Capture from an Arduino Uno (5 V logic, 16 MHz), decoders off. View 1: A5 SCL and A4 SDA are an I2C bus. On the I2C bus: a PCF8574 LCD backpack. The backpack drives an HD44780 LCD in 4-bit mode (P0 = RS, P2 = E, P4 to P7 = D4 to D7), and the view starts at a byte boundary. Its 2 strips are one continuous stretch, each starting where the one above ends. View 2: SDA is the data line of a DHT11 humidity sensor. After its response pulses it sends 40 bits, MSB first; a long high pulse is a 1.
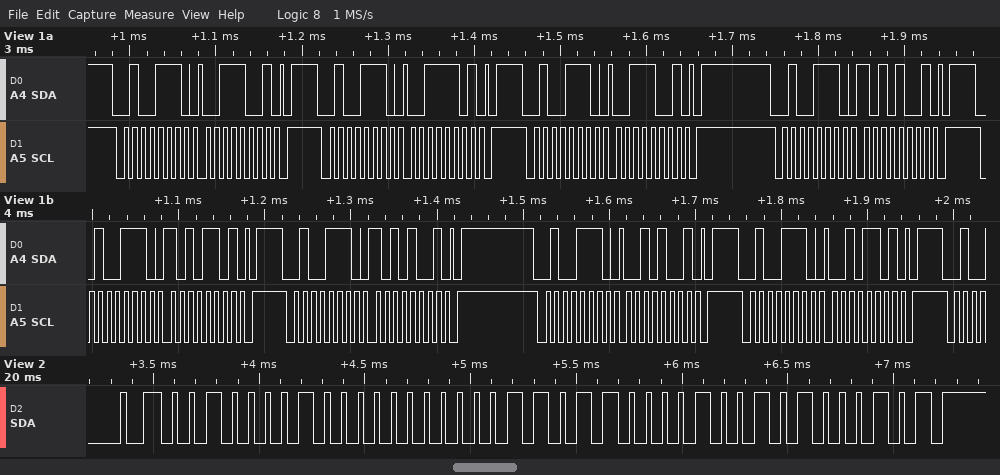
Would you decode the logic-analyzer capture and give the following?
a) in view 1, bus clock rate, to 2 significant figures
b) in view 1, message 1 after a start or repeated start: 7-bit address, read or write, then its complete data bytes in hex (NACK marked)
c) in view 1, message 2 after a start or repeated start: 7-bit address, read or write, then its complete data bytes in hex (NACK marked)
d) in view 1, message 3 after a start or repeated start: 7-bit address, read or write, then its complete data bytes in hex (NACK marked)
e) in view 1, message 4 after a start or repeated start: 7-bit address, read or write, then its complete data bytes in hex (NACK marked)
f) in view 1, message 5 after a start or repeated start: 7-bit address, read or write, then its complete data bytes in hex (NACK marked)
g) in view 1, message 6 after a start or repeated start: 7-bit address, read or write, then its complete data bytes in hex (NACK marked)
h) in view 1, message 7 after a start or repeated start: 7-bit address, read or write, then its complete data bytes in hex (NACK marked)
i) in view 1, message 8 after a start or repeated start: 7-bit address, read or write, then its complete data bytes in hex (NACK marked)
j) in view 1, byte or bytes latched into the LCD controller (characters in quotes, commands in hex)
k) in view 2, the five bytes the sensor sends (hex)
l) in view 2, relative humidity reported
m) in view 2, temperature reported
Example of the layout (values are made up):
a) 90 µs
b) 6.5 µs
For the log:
a) 100 kHz
b) 0x27 write: 39
c) 0x27 write: 3D
d) 0x27 write: 39
e) 0x27 write: A9
f) 0x27 write: AD
g) 0x27 write: A9
h) 0x27 write: 29
i) 0x27 write: 2D
j) ':'
k) 21 00 1B 09 45
l) 33 %
m) 27.9 °C
